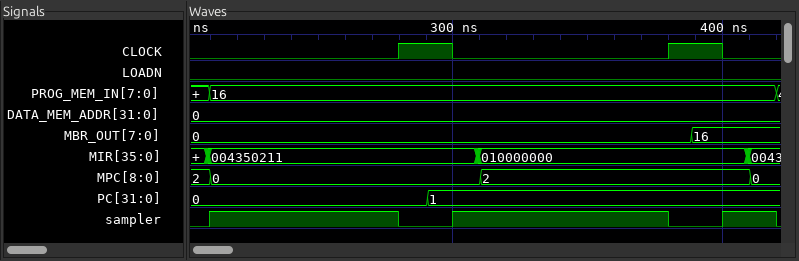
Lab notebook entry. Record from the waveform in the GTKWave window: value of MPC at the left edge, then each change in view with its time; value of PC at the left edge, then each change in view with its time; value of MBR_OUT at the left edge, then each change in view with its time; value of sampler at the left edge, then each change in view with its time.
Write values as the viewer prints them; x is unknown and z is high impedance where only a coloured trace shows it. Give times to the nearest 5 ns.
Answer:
2, 0 at 210 ns, 2 at 310 ns, 0 at 410 ns
0, 1 at 290 ns
0, 16 at 390 ns
0, 1 at 210 ns, 0 at 280 ns, 1 at 300 ns, 0 at 380 ns, 1 at 400 ns, 0 at 420 ns
